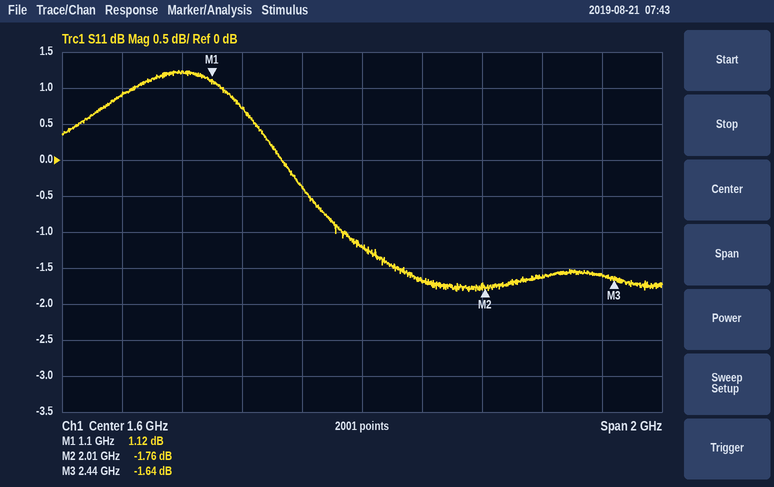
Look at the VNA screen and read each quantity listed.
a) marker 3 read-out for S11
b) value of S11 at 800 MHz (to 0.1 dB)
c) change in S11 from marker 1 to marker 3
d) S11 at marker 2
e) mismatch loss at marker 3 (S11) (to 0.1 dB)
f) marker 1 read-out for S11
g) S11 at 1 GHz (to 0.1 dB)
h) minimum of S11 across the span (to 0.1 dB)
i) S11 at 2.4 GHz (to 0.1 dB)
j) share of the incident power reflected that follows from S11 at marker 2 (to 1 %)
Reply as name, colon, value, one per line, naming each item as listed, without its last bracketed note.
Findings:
marker 3 read-out for S11: -1.64 dB
value of S11 at 800 MHz: 0.9 dB
change in S11 from marker 1 to marker 3: -2.76 dB
S11 at marker 2: -1.76 dB
mismatch loss at marker 3 (S11): 5.0 dB
marker 1 read-out for S11: 1.12 dB
S11 at 1 GHz: 1.2 dB
minimum of S11 across the span: -1.8 dB
S11 at 2.4 GHz: -1.6 dB
share of the incident power reflected that follows from S11 at marker 2: 67 %
